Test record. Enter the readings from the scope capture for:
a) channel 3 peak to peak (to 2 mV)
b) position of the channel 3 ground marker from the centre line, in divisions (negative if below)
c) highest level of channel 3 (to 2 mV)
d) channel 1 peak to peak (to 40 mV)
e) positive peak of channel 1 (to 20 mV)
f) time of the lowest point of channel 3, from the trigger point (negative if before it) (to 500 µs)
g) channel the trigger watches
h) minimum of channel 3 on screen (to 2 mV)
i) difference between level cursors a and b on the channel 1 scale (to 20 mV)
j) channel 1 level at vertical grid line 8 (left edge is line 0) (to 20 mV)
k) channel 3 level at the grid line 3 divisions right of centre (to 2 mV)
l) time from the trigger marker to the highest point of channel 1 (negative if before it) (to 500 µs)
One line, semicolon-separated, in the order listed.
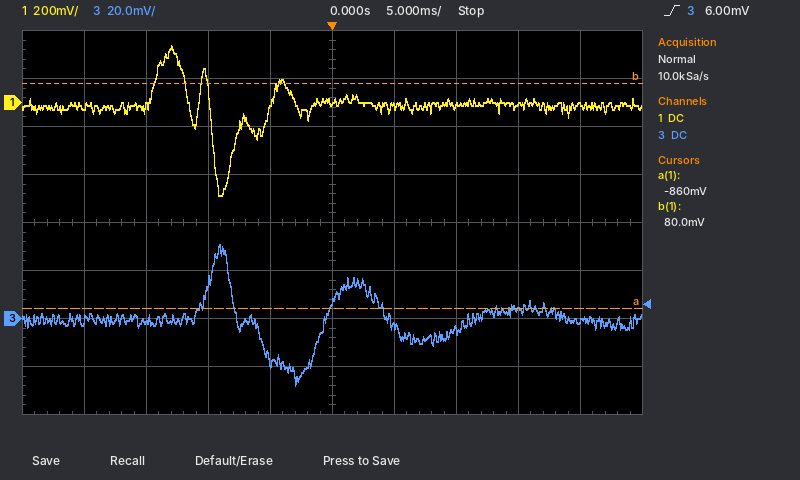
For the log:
58 mV; -2.0 div; 30 mV; 640 mV; 240 mV; -3.0 ms; channel 3; -28 mV; 940 mV; 0 mV; 4 mV; -13.0 ms
